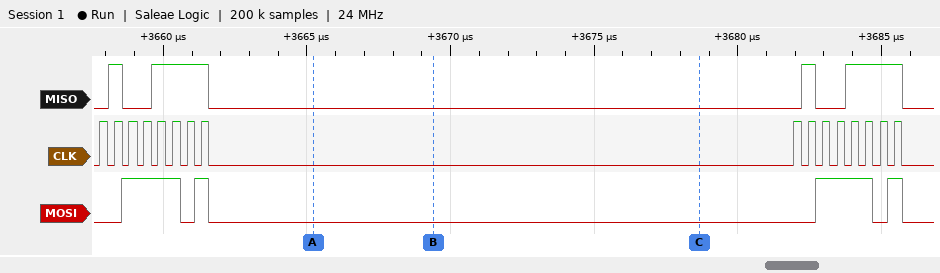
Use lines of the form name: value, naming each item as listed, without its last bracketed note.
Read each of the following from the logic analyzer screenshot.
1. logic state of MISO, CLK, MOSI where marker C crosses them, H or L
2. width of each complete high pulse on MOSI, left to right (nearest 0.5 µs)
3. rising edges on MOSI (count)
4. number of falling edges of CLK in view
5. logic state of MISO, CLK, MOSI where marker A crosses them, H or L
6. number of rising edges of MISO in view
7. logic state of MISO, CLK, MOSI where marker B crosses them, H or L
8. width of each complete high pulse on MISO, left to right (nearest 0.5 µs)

logic state of MISO, CLK, MOSI where marker C crosses them, H or L: MISO=L, CLK=L, MOSI=L
width of each complete high pulse on MOSI, left to right: 2 µs, 0.5 µs, 2 µs, 0.5 µs
rising edges on MOSI: 4
number of falling edges of CLK in view: 16
logic state of MISO, CLK, MOSI where marker A crosses them, H or L: MISO=L, CLK=L, MOSI=L
number of rising edges of MISO in view: 4
logic state of MISO, CLK, MOSI where marker B crosses them, H or L: MISO=L, CLK=L, MOSI=L
width of each complete high pulse on MISO, left to right: 0.5 µs, 2 µs, 0.5 µs, 2 µs
